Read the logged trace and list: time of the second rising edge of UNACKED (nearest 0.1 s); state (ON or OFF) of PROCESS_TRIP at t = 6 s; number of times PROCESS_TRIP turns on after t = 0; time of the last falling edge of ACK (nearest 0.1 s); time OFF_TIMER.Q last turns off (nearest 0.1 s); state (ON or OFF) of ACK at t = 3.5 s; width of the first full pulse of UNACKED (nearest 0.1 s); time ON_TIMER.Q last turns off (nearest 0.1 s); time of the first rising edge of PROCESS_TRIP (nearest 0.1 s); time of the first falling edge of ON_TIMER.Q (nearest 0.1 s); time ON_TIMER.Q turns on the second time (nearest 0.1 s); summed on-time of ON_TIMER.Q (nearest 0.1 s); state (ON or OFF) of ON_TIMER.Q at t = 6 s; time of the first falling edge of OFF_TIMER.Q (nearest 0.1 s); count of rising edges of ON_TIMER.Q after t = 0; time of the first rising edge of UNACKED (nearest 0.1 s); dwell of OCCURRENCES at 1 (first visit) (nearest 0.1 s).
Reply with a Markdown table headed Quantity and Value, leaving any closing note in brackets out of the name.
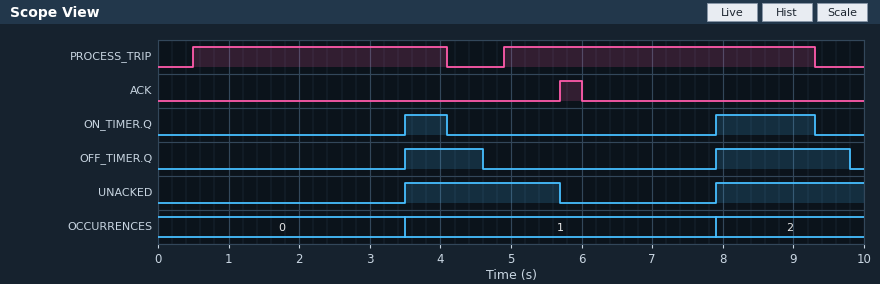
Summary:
| Quantity | Value |
|---|---|
| time of the second rising edge of UNACKED | 7.9 s |
| state (ON or OFF) of PROCESS_TRIP at t = 6 s | ON |
| number of times PROCESS_TRIP turns on after t = 0 | 2 |
| time of the last falling edge of ACK | 6.0 s |
| time OFF_TIMER.Q last turns off | 9.8 s |
| state (ON or OFF) of ACK at t = 3.5 s | OFF |
| width of the first full pulse of UNACKED | 2.2 s |
| time ON_TIMER.Q last turns off | 9.3 s |
| time of the first rising edge of PROCESS_TRIP | 0.5 s |
| time of the first falling edge of ON_TIMER.Q | 4.1 s |
| time ON_TIMER.Q turns on the second time | 7.9 s |
| summed on-time of ON_TIMER.Q | 2.0 s |
| state (ON or OFF) of ON_TIMER.Q at t = 6 s | OFF |
| time of the first falling edge of OFF_TIMER.Q | 4.6 s |
| count of rising edges of ON_TIMER.Q after t = 0 | 2 |
| time of the first rising edge of UNACKED | 3.5 s |
| dwell of OCCURRENCES at 1 (first visit) | 4.4 s |
